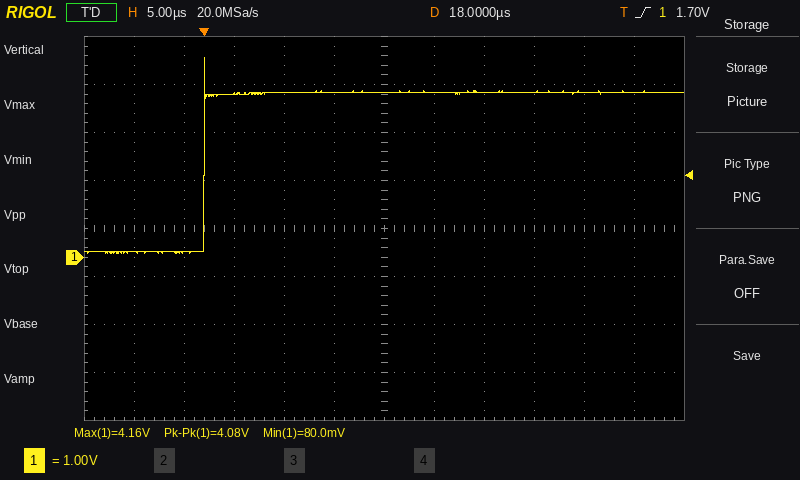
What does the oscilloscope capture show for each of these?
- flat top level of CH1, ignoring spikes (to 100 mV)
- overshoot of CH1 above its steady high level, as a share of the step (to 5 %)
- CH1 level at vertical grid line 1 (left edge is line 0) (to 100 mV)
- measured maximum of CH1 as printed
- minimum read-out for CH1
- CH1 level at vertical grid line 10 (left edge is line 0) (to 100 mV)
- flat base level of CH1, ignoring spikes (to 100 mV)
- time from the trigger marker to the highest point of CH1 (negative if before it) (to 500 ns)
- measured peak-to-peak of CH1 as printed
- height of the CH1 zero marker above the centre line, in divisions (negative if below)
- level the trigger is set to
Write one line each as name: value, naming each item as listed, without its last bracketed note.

flat top level of CH1, ignoring spikes: 3.4 V
overshoot of CH1 above its steady high level, as a share of the step: 20 %
CH1 level at vertical grid line 1 (left edge is line 0): 100 mV
measured maximum of CH1 as printed: 4.16 V
minimum read-out for CH1: 80.0 mV
CH1 level at vertical grid line 10 (left edge is line 0): 3.4 V
flat base level of CH1, ignoring spikes: 100 mV
time from the trigger marker to the highest point of CH1 (negative if before it): 0.0 µs
measured peak-to-peak of CH1 as printed: 4.08 V
height of the CH1 zero marker above the centre line, in divisions: -0.6 div
level the trigger is set to: 1.70 V
